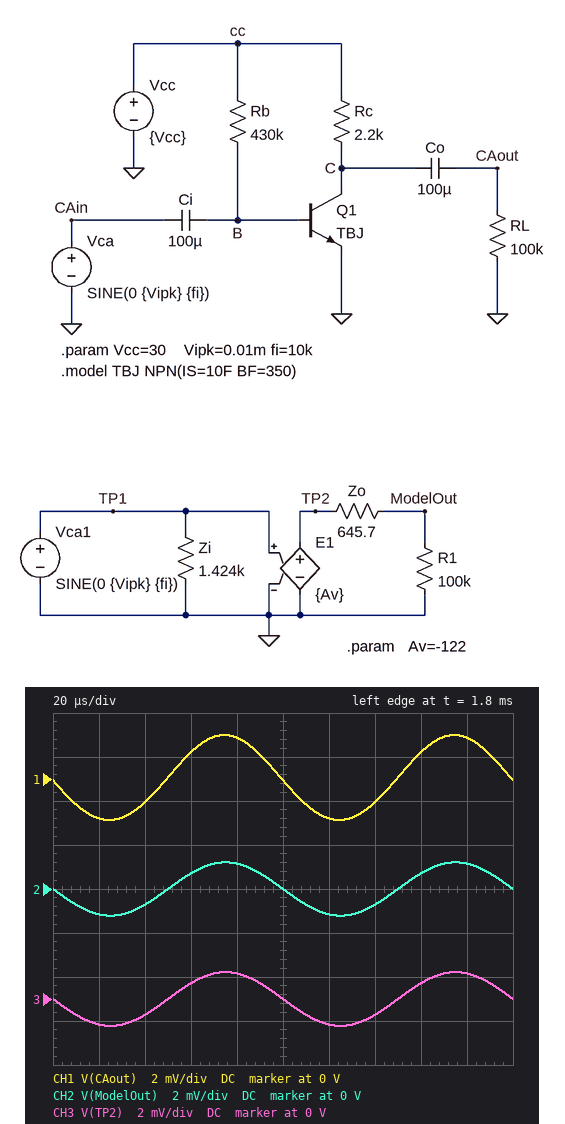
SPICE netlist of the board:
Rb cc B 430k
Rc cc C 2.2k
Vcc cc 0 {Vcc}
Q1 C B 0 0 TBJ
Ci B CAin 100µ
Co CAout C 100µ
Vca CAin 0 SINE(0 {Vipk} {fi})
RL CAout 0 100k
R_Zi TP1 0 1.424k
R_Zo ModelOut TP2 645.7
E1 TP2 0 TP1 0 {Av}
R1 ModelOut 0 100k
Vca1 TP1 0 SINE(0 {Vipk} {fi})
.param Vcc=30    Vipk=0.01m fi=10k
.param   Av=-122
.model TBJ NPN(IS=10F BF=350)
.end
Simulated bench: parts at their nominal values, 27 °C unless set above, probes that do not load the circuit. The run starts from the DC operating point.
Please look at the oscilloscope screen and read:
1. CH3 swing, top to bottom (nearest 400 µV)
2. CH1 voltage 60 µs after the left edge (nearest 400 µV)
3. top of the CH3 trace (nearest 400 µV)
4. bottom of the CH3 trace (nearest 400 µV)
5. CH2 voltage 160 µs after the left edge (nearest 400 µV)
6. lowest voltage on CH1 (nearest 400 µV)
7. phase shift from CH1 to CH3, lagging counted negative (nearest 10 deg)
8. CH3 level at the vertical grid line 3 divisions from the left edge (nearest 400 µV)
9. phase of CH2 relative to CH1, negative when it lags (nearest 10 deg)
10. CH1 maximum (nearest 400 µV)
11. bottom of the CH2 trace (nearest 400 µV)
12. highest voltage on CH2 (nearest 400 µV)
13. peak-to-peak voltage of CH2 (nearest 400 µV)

2.4 mV
1.2 mV
1.2 mV
-1.2 mV
800 µV
-2.0 mV
0 deg
800 µV
0 deg
2.0 mV
-1.2 mV
1.2 mV
2.4 mV
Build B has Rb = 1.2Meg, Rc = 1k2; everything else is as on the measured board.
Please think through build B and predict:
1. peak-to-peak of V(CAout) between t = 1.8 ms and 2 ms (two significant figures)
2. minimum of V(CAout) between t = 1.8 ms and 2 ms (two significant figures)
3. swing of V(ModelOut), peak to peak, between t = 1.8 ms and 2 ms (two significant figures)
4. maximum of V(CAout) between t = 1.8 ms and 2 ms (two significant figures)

7.8 mV
-3.9 mV
2.4 mV
3.9 mV
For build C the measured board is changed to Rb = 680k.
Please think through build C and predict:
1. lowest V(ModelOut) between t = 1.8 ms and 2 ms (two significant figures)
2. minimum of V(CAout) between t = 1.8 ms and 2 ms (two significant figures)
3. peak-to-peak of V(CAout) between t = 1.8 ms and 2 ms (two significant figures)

-1.2 mV
-6.0 mV
13 mV
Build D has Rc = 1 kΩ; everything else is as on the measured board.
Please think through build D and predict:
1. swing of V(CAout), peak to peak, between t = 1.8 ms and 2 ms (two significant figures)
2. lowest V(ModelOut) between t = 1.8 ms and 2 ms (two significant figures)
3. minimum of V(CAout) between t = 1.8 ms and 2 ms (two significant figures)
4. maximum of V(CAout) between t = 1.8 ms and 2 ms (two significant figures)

18 mV
-1.2 mV
-9.1 mV
9.1 mV
